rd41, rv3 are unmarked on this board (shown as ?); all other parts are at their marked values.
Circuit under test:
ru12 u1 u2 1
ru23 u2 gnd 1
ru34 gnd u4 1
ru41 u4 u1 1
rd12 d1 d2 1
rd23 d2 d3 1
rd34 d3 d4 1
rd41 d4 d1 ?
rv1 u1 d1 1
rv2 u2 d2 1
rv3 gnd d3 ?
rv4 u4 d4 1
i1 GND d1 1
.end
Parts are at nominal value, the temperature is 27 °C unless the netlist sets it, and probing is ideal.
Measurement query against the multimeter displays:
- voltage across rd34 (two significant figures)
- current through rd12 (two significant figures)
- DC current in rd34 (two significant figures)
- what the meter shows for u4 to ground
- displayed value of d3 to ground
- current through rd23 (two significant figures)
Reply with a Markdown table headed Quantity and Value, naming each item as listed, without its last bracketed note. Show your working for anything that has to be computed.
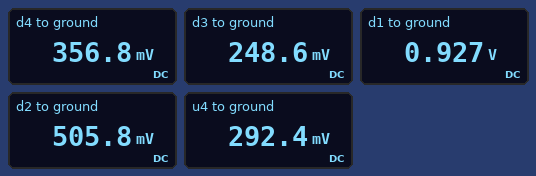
| Quantity | Value |
|---|---|
| voltage across rd34 | 356.8 mV - 248.6 mV = 110 mV |
| current through rd12 | (927 mV - 505.8 mV) / 1 Ω = 420 mA |
| DC current in rd34 | (356.8 mV - 248.6 mV) / 1 Ω = 110 mA |
| what the meter shows for u4 to ground | 292.4 mV |
| displayed value of d3 to ground | 248.6 mV |
| current through rd23 | (505.8 mV - 248.6 mV) / 1 Ω = 260 mA |
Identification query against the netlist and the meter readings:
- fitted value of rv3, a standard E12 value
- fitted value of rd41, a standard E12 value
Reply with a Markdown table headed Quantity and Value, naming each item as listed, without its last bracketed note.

| Quantity | Value |
|---|---|
| fitted value of rv3, a standard E12 value | 0.68 Ω |
| fitted value of rd41, a standard E12 value | 3.3 Ω |
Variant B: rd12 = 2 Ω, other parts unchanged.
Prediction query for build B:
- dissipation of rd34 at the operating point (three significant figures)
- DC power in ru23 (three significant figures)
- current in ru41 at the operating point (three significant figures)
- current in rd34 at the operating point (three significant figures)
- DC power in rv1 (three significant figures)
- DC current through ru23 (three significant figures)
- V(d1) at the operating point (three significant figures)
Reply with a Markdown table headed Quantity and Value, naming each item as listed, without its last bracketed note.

| Quantity | Value |
|---|---|
| dissipation of rd34 at the operating point | 20.4 mW |
| DC power in ru23 | 113 mW |
| current in ru41 at the operating point | 254 mA |
| current in rd34 at the operating point | 143 mA |
| DC power in rv1 | 237 mW |
| DC current through ru23 | 337 mA |
| V(d1) at the operating point | 1.06 V |
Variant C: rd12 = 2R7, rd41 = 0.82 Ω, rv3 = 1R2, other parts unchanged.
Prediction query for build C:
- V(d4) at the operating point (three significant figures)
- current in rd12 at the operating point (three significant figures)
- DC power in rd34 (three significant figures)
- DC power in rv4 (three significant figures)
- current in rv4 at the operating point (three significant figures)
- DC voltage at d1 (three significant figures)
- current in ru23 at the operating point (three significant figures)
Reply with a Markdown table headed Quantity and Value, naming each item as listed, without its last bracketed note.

| Quantity | Value |
|---|---|
| V(d4) at the operating point | 581 mV |
| current in rd12 at the operating point | 184 mA |
| DC power in rd34 | 49.5 mW |
| DC power in rv4 | 42.3 mW |
| current in rv4 at the operating point | 206 mA |
| DC voltage at d1 | 932 mV |
| current in ru23 at the operating point | 326 mA |
